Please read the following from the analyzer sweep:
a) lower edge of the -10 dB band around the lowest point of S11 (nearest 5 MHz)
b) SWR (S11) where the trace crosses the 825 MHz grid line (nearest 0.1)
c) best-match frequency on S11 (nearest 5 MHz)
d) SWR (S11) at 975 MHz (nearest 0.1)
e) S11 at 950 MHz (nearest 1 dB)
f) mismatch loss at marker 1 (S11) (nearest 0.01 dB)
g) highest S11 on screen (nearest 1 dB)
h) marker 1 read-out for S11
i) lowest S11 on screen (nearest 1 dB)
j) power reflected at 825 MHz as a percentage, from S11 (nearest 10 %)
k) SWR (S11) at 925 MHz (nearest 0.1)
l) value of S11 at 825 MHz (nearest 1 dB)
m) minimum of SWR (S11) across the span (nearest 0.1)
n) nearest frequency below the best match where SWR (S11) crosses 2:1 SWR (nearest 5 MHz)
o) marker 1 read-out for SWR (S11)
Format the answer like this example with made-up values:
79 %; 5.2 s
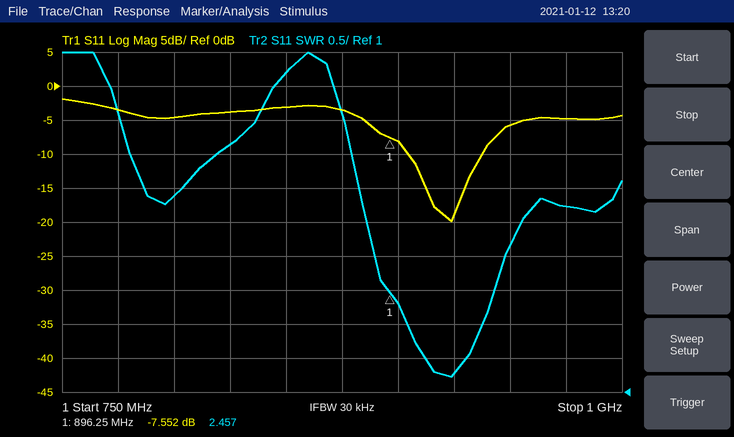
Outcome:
905 MHz; 4.6; 925 MHz; 3.7; -6 dB; 0.84 dB; -2 dB; -7.552 dB; -20 dB; 40 %; 1.3; -4 dB; 1.2; 905 MHz; 2.457
